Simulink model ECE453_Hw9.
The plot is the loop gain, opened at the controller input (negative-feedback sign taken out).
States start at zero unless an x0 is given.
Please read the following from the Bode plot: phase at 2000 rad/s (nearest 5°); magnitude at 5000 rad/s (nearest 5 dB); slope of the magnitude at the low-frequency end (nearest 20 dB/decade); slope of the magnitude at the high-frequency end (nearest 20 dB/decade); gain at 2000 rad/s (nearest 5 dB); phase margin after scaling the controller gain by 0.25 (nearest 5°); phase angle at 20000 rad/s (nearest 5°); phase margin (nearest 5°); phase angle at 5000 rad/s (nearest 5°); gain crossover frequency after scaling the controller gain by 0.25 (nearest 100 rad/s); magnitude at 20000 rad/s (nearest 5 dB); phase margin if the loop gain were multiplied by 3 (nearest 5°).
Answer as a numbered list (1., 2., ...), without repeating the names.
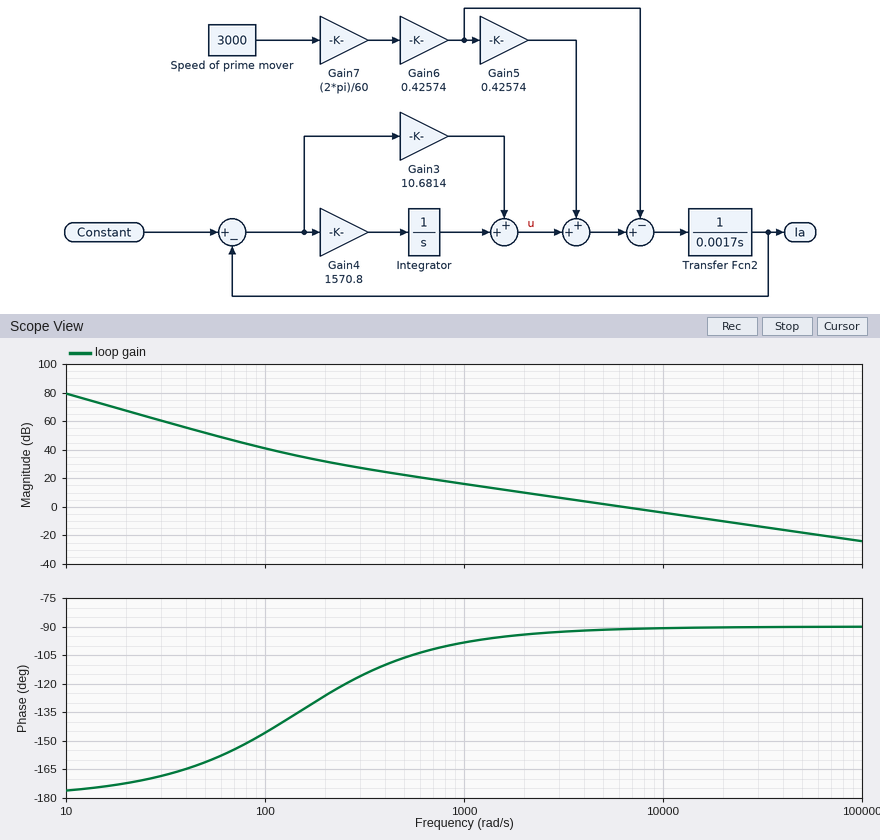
1. -95°
2. 0 dB
3. -40 dB/decade
4. -20 dB/decade
5. 10 dB
6. 85°
7. -90°
8. 90°
9. -90°
10. 1600 rad/s
11. -10 dB
12. 90°
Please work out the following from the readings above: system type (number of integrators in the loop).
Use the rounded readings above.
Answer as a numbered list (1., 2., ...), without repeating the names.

1. 2
